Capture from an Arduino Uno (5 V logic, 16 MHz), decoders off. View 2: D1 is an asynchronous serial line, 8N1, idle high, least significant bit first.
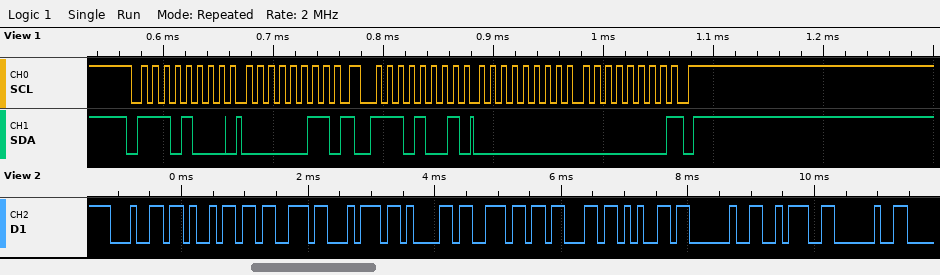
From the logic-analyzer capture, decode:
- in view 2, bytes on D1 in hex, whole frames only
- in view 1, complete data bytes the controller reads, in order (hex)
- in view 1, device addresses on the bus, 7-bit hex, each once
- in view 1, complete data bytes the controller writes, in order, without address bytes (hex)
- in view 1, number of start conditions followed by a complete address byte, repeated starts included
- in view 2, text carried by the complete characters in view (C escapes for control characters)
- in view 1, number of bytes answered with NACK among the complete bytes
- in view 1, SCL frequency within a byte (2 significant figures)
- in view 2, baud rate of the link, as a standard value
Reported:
64 69 73 74 61 6E 63 65 20 3A 20
00 00
0x74
03
2
"distance : "
1
100 kHz
9600 baud
